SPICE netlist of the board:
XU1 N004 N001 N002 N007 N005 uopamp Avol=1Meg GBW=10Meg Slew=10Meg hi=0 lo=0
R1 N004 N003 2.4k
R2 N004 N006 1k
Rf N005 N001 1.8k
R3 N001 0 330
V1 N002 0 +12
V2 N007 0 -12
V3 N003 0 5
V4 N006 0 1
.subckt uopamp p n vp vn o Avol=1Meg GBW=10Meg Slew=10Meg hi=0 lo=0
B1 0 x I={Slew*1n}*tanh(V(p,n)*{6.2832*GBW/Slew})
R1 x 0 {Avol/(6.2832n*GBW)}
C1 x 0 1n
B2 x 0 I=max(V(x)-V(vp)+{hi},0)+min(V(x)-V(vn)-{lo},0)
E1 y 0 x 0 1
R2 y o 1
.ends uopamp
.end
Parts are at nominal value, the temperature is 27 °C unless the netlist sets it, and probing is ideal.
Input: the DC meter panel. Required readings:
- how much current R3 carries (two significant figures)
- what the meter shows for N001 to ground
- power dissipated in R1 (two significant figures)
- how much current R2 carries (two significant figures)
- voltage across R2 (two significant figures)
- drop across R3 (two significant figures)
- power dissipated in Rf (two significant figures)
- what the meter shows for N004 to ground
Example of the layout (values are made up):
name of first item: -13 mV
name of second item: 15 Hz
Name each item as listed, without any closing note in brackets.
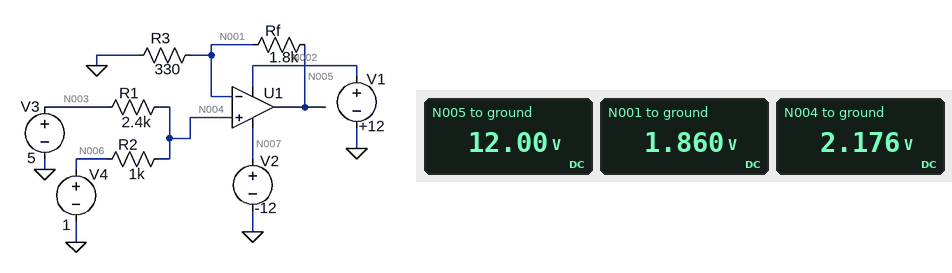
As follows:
how much current R3 carries: 5.6 mA
what the meter shows for N001 to ground: 1.860 V
power dissipated in R1: 3.3 mW
how much current R2 carries: 1.2 mA
voltage across R2: 1.2 V
drop across R3: 1.9 V
power dissipated in Rf: 57 mW
what the meter shows for N004 to ground: 2.176 V
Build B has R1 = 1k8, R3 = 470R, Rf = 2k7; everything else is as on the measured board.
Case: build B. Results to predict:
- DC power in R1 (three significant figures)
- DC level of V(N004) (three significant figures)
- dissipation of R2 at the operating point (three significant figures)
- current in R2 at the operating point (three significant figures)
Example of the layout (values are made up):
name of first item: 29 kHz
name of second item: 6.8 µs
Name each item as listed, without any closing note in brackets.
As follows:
DC power in R1: 3.67 mW
DC level of V(N004): 2.43 V
dissipation of R2 at the operating point: 2.04 mW
current in R2 at the operating point: 1.43 mA
